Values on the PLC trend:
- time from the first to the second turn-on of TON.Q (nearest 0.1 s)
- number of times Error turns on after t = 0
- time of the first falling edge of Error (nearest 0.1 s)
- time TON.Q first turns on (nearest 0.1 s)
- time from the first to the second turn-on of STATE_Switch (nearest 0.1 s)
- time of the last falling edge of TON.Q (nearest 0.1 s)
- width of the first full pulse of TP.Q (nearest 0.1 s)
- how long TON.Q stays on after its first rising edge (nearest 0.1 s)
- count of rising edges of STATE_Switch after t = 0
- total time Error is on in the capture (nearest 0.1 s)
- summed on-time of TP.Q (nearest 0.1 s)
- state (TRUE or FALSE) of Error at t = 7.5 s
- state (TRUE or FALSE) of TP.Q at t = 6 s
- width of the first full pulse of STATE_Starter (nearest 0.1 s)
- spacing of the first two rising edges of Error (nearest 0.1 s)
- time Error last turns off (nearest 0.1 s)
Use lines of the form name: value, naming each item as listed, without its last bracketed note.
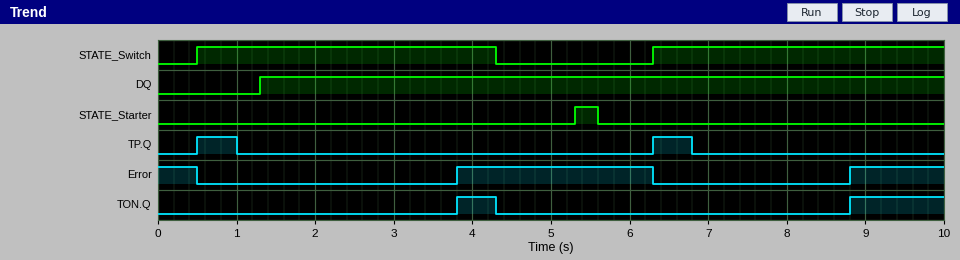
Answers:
time from the first to the second turn-on of TON.Q: 5.0 s
number of times Error turns on after t = 0: 2
time of the first falling edge of Error: 0.5 s
time TON.Q first turns on: 3.8 s
time from the first to the second turn-on of STATE_Switch: 5.8 s
time of the last falling edge of TON.Q: 4.3 s
width of the first full pulse of TP.Q: 0.5 s
how long TON.Q stays on after its first rising edge: 0.5 s
count of rising edges of STATE_Switch after t = 0: 2
total time Error is on in the capture: 4.2 s
summed on-time of TP.Q: 1.0 s
state (TRUE or FALSE) of Error at t = 7.5 s: FALSE
state (TRUE or FALSE) of TP.Q at t = 6 s: FALSE
width of the first full pulse of STATE_Starter: 0.3 s
spacing of the first two rising edges of Error: 5.0 s
time Error last turns off: 6.3 s
